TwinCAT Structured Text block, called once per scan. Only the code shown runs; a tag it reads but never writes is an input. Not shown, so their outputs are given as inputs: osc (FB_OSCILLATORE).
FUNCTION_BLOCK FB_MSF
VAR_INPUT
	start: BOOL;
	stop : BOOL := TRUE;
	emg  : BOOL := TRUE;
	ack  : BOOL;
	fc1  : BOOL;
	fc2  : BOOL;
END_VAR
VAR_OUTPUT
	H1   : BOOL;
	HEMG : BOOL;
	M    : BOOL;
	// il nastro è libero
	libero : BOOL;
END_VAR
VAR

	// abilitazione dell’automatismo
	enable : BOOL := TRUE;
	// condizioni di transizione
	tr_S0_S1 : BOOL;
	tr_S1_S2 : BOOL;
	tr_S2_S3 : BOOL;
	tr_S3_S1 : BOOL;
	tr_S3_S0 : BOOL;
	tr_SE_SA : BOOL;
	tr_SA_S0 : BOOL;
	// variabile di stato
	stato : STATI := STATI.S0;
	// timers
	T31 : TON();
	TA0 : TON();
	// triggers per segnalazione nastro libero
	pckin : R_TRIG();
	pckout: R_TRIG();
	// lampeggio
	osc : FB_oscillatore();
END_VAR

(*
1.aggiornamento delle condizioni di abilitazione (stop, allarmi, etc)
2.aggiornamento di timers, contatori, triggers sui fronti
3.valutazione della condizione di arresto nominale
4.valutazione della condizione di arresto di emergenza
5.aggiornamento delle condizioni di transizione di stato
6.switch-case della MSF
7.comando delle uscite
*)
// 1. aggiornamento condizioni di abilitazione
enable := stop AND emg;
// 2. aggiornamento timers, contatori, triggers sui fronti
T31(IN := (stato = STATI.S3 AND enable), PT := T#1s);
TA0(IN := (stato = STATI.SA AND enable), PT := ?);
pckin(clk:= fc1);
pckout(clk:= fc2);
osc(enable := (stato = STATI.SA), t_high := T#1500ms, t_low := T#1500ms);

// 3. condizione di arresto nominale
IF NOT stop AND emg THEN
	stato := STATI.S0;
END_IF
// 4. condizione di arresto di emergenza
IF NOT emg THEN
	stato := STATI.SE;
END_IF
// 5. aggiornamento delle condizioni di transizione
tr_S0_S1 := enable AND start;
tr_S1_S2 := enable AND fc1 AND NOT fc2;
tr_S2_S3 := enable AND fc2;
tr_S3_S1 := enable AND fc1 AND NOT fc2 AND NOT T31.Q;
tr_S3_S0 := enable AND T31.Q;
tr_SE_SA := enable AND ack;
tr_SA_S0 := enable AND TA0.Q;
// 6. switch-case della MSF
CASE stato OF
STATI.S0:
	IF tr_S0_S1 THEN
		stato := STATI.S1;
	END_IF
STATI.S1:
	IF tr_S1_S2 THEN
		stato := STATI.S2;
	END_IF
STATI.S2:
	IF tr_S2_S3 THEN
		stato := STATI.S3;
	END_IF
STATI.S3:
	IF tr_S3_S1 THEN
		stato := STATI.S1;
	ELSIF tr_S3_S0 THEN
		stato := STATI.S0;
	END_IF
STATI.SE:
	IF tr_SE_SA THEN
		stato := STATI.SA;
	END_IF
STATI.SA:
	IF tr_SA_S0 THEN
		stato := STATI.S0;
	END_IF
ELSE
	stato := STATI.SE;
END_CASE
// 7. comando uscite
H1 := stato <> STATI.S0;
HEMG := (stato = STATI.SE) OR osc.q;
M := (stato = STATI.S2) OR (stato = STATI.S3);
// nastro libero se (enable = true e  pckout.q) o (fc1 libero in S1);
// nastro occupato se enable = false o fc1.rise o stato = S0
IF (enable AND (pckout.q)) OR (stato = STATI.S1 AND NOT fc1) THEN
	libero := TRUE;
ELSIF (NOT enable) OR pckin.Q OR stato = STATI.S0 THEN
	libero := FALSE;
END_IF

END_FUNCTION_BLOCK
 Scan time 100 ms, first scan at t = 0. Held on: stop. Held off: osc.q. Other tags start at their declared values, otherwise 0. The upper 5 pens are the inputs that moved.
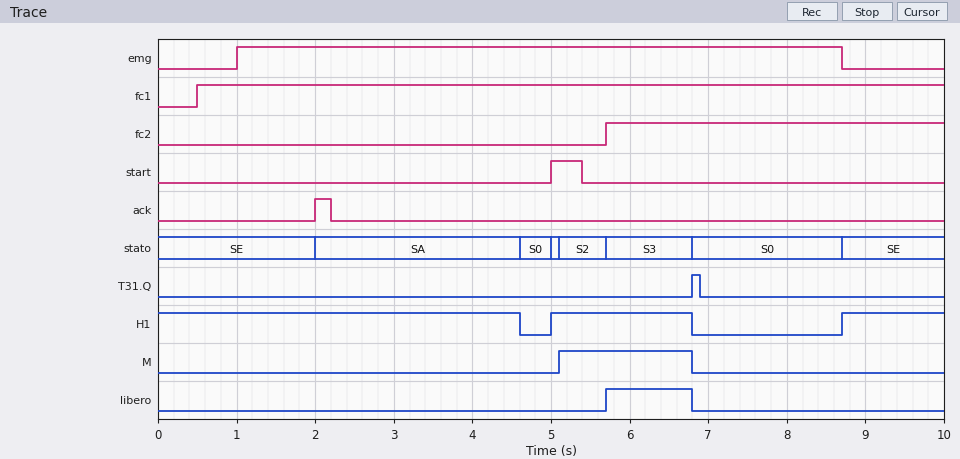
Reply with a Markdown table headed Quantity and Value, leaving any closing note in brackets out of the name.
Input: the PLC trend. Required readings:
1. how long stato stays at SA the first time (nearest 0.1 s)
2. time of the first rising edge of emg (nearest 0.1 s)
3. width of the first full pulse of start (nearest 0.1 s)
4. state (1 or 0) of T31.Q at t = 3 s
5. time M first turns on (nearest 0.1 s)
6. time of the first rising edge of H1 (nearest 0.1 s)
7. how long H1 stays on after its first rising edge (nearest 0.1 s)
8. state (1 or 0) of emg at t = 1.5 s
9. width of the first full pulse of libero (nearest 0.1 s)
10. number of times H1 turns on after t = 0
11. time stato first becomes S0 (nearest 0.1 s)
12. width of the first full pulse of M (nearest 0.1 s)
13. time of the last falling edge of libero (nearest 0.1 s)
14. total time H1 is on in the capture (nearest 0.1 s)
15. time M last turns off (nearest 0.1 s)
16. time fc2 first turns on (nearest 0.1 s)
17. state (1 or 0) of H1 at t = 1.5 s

| Quantity | Value |
|---|---|
| how long stato stays at SA the first time | 2.6 s |
| time of the first rising edge of emg | 1.0 s |
| width of the first full pulse of start | 0.4 s |
| state (1 or 0) of T31.Q at t = 3 s | 0 |
| time M first turns on | 5.1 s |
| time of the first rising edge of H1 | 5.0 s |
| how long H1 stays on after its first rising edge | 1.8 s |
| state (1 or 0) of emg at t = 1.5 s | 1 |
| width of the first full pulse of libero | 1.1 s |
| number of times H1 turns on after t = 0 | 2 |
| time stato first becomes S0 | 4.6 s |
| width of the first full pulse of M | 1.7 s |
| time of the last falling edge of libero | 6.8 s |
| total time H1 is on in the capture | 7.7 s |
| time M last turns off | 6.8 s |
| time fc2 first turns on | 5.7 s |
| state (1 or 0) of H1 at t = 1.5 s | 1 |
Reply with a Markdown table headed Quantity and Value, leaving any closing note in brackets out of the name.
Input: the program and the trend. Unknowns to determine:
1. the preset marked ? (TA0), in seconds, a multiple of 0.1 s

| Quantity | Value |
|---|---|
| the preset marked ? (TA0), in seconds, a multiple of 0.1 s | 2.5 s |
